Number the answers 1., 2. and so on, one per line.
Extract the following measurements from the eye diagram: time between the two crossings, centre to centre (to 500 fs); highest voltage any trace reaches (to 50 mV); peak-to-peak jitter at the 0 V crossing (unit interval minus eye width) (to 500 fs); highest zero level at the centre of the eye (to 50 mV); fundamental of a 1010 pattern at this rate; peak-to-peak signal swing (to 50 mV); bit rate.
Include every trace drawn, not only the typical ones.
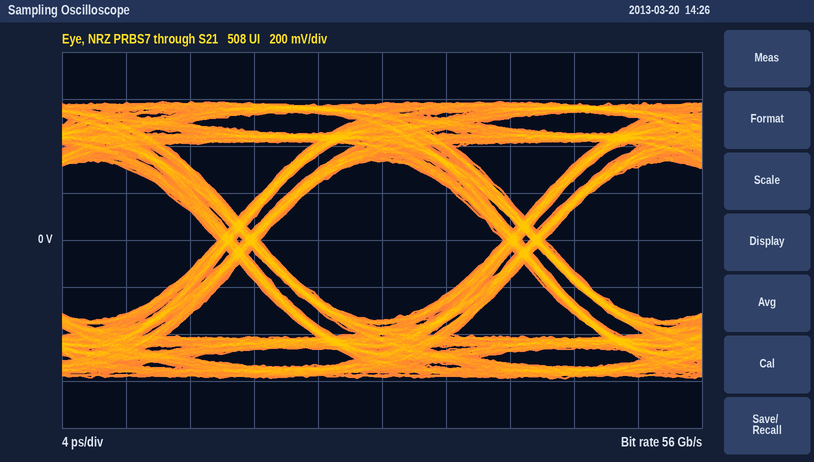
1. 18.0 ps
2. 600 mV
3. 2.5 ps
4. -350 mV
5. 28 GHz
6. 1.20 V
7. 56 Gb/s
